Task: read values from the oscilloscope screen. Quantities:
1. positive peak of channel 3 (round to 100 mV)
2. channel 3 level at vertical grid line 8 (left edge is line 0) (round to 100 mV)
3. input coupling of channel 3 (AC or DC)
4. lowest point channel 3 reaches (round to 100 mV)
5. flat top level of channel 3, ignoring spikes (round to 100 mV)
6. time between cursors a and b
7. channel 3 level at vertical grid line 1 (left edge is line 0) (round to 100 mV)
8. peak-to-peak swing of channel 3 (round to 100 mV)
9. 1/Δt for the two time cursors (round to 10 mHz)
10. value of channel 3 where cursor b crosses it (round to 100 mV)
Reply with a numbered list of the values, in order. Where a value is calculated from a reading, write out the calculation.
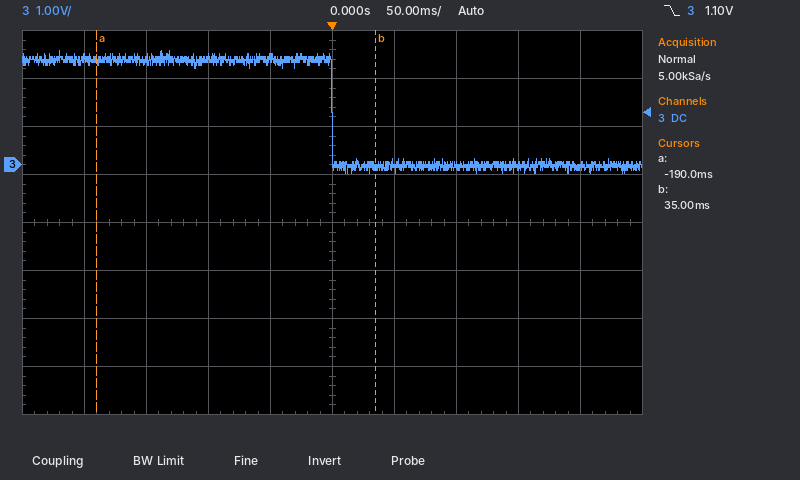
1. 2.4 V
2. 0.0 V
3. DC
4. -200 mV
5. 2.2 V
6. 35 ms − (-190 ms) = 225 ms
7. 2.2 V
8. 2.4 V − (-200 mV) = 2.6 V
9. 1 / 225 ms ≈ 4.44 Hz
10. 0.0 V
